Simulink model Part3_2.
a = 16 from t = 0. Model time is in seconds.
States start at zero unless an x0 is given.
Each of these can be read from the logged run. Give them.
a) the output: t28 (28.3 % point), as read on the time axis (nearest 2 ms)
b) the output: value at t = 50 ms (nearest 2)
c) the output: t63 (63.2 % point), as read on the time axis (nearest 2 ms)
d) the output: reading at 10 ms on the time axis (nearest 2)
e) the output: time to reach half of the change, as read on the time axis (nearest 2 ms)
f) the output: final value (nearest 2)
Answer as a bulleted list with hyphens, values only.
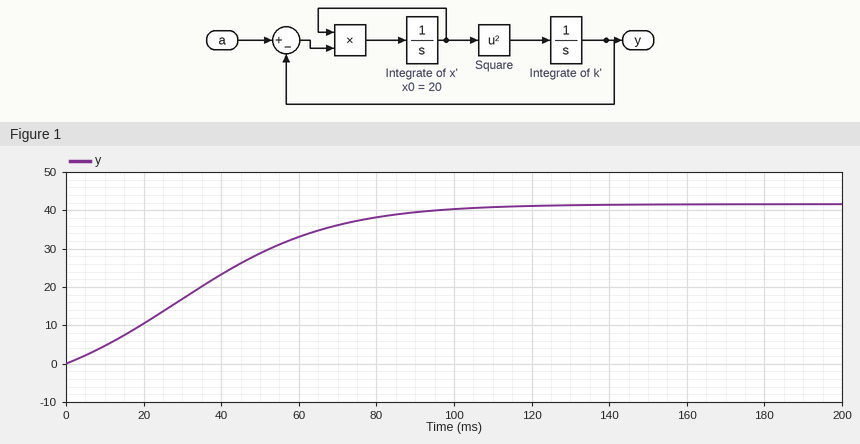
- 22 ms
- 28
- 46 ms
- 4
- 36 ms
- 42
